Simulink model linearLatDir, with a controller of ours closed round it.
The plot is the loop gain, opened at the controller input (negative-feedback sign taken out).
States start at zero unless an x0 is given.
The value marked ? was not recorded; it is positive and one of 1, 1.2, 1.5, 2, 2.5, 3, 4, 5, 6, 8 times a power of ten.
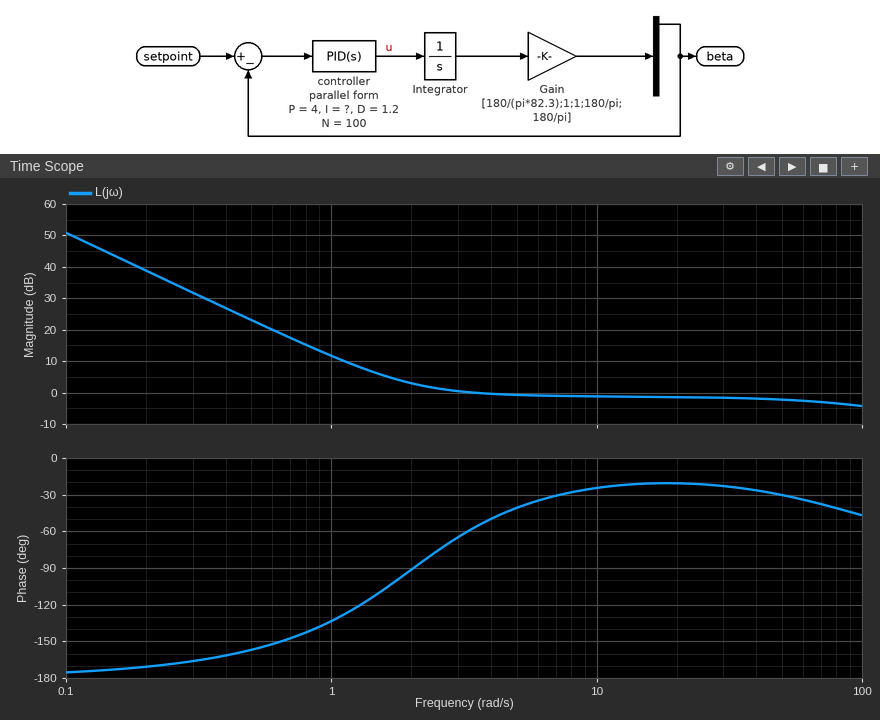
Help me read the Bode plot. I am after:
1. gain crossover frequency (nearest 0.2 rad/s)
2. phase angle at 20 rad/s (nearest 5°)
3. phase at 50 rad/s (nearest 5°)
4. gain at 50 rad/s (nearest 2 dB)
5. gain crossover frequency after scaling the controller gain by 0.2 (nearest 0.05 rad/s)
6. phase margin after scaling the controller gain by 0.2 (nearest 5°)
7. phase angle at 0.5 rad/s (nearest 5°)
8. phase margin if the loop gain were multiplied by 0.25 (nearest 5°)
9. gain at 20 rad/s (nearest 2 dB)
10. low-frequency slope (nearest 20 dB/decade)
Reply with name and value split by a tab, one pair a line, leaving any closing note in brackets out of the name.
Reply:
gain crossover frequency	3.4 rad/s
phase angle at 20 rad/s	-20°
phase at 50 rad/s	-30°
gain at 50 rad/s	-2 dB
gain crossover frequency after scaling the controller gain by 0.2	0.85 rad/s
phase margin after scaling the controller gain by 0.2	40°
phase angle at 0.5 rad/s	-155°
phase margin if the loop gain were multiplied by 0.25	45°
gain at 20 rad/s	-2 dB
low-frequency slope	-40 dB/decade
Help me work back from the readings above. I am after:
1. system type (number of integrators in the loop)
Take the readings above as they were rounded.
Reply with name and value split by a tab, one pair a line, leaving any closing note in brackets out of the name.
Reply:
system type	2
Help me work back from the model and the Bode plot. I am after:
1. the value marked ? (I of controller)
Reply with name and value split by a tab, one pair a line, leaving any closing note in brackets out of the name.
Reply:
the value marked ?	5
